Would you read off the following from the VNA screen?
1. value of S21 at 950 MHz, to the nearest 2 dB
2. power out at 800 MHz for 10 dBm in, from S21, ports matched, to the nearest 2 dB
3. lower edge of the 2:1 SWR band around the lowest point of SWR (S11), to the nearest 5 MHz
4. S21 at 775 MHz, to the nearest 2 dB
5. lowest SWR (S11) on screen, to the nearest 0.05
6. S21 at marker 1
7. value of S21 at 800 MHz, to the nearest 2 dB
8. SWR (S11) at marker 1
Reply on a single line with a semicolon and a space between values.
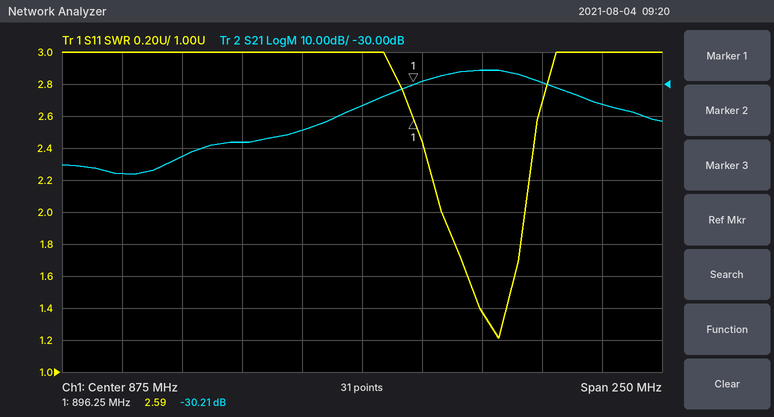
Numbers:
-30 dB; -42 dBm; 910 MHz; -58 dB; 1.20; -30.21 dB; -52 dB; 2.59
